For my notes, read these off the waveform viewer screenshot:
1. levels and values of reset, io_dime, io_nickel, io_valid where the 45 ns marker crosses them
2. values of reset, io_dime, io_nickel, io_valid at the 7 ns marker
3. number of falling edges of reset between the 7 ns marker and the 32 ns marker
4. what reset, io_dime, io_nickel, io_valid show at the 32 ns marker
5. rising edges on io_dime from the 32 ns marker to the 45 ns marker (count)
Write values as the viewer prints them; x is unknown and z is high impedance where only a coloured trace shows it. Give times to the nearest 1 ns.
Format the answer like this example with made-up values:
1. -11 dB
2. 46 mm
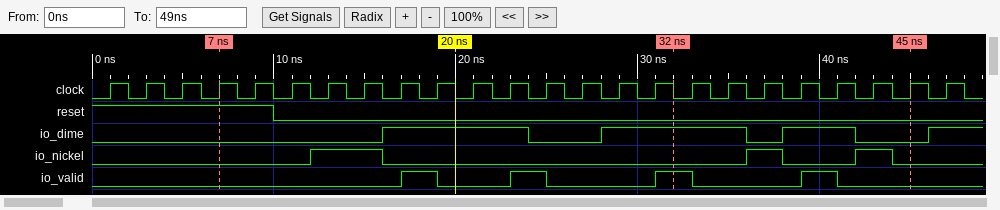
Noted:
1. reset=0, io_dime=0, io_nickel=0, io_valid=0
2. reset=1, io_dime=0, io_nickel=0, io_valid=0
3. 1
4. reset=0, io_dime=1, io_nickel=0, io_valid=1
5. 1
